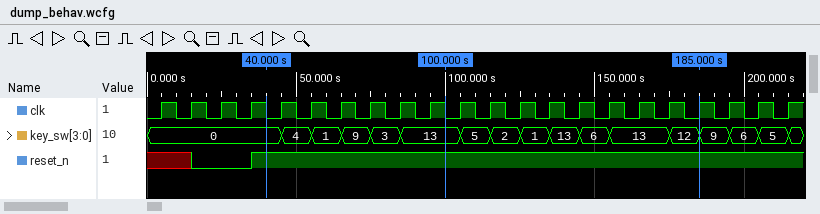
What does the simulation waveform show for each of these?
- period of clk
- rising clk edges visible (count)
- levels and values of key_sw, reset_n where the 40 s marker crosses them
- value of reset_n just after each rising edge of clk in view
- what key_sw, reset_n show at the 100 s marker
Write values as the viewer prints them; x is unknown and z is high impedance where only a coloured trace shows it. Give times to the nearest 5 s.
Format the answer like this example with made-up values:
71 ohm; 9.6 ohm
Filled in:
10 s; 22; key_sw=0, reset_n=1; x 0 0 1 1 1 1 1 1 1 1 1 1 1 1 1 1 1 1 1 1 1; key_sw=13, reset_n=1
